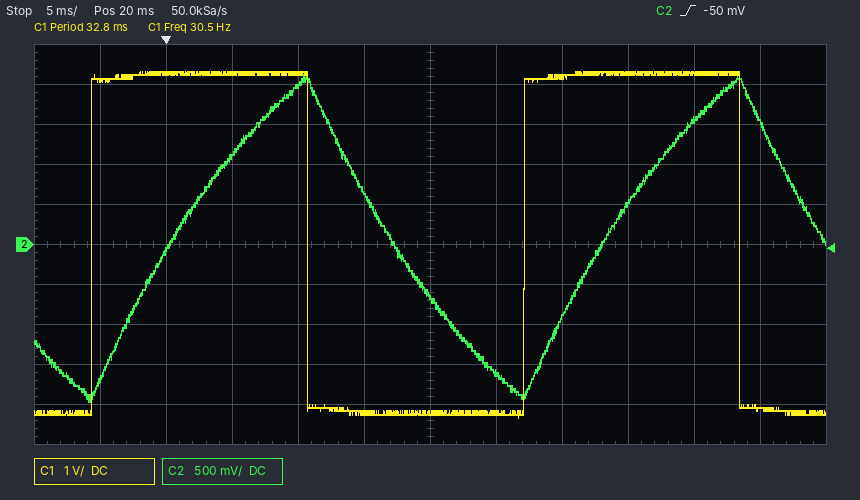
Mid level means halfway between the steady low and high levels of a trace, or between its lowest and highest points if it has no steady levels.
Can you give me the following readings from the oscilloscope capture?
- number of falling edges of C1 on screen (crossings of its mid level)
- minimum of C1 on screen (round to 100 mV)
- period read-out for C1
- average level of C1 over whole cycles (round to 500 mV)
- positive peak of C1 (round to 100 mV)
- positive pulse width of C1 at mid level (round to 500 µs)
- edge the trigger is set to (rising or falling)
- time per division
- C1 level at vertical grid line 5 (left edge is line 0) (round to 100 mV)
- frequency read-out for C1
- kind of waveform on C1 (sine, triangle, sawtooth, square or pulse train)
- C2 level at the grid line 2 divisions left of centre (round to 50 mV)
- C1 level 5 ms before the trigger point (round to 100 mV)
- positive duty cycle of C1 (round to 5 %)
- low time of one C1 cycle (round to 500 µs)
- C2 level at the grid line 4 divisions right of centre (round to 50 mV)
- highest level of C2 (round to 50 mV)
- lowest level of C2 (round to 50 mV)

2
-4.3 V
32.8 ms
0.0 V
4.3 V
16.5 ms
rising
5 ms
-4.2 V
30.5 Hz
square
2.00 V
4.1 V
50 %
16.5 ms
1.55 V
2.10 V
-1.95 V
